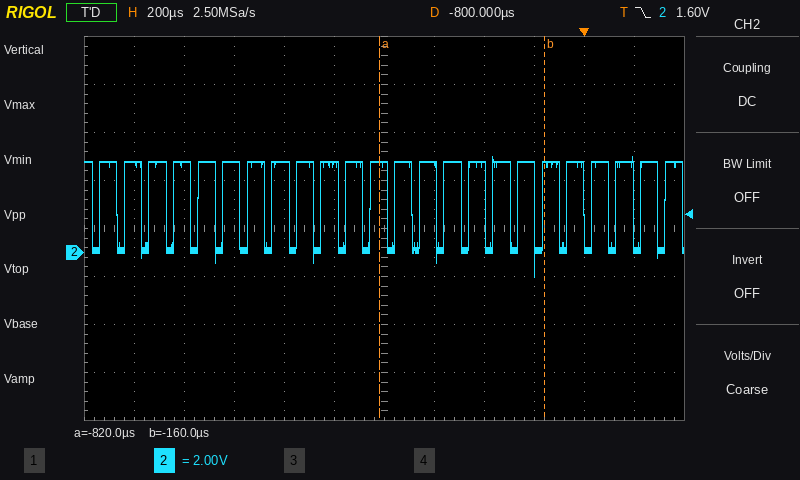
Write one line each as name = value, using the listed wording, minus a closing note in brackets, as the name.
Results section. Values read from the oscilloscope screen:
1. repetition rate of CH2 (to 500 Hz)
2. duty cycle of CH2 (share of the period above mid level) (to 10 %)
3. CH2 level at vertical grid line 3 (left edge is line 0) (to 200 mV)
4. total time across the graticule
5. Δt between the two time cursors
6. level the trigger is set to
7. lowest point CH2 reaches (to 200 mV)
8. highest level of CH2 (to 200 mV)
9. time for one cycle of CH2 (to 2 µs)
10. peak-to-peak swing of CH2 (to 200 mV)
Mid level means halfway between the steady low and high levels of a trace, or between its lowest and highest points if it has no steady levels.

repetition rate of CH2 = 10.0 kHz
duty cycle of CH2 (share of the period above mid level) = 70 %
CH2 level at vertical grid line 3 (left edge is line 0) = 3.8 V
total time across the graticule = 2.4 ms
Δt between the two time cursors = 660 µs
level the trigger is set to = 1.60 V
lowest point CH2 reaches = -1.0 V
highest level of CH2 = 4.0 V
time for one cycle of CH2 = 98 µs
peak-to-peak swing of CH2 = 5.0 V
